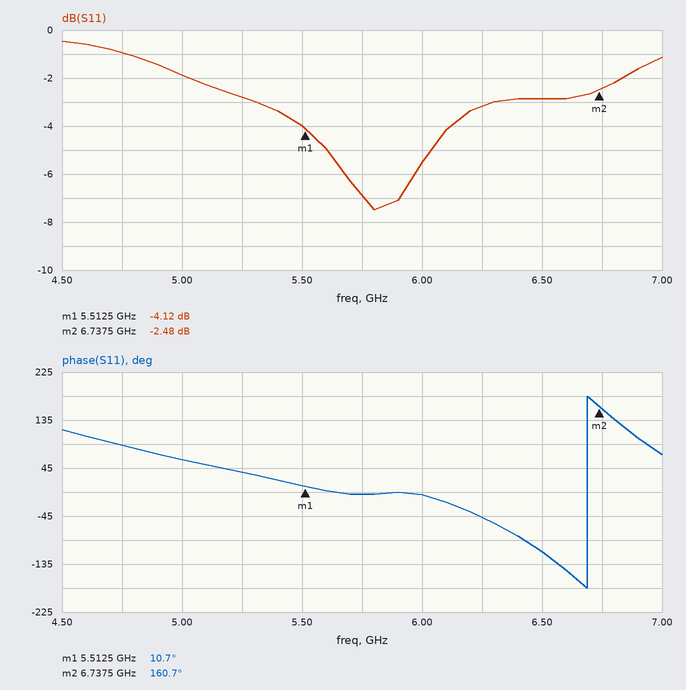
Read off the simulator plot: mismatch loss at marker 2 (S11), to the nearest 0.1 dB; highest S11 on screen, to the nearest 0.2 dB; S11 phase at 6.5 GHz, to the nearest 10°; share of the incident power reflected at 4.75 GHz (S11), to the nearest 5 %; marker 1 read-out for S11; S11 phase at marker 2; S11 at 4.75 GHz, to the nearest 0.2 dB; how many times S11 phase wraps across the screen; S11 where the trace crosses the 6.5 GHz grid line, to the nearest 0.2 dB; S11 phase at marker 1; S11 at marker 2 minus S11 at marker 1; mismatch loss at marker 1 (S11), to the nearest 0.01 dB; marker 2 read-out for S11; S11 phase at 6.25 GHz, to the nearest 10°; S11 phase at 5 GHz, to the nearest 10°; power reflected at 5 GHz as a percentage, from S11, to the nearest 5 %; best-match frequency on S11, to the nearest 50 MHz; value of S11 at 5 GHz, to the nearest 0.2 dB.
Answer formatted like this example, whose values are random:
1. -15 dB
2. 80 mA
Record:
1. 3.6 dB
2. -0.4 dB
3. -110°
4. 80 %
5. -4.12 dB
6. 160.7°
7. -1.0 dB
8. 1
9. -2.8 dB
10. 10.7°
11. 1.64 dB
12. 2.13 dB
13. -2.48 dB
14. -50°
15. 60°
16. 65 %
17. 5.80 GHz
18. -1.8 dB
